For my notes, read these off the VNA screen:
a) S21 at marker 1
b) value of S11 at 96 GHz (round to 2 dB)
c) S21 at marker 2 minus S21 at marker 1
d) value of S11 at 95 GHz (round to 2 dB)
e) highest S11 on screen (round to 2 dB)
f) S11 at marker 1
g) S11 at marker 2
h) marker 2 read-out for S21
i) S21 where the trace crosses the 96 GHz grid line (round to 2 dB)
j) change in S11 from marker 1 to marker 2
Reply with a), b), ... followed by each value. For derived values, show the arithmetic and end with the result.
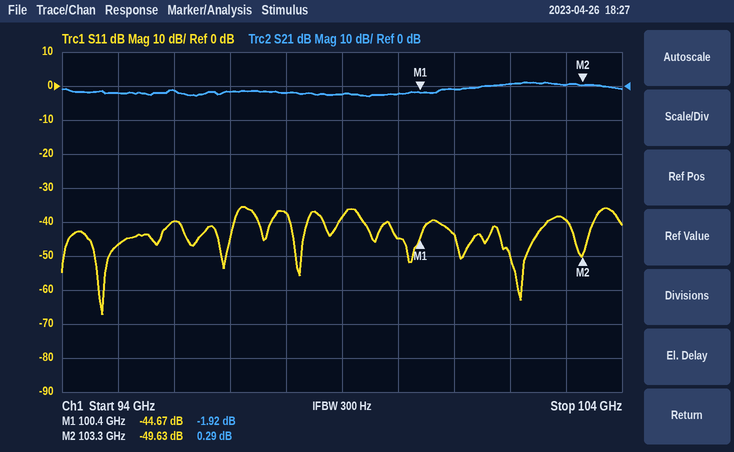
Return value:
a) -1.92 dB
b) -40 dB
c) 0.29 − (-1.92) = 2.21 dB
d) -46 dB
e) -36 dB
f) -44.67 dB
g) -49.63 dB
h) 0.29 dB
i) -2 dB
j) -49.63 − (-44.67) = -4.96 dB
